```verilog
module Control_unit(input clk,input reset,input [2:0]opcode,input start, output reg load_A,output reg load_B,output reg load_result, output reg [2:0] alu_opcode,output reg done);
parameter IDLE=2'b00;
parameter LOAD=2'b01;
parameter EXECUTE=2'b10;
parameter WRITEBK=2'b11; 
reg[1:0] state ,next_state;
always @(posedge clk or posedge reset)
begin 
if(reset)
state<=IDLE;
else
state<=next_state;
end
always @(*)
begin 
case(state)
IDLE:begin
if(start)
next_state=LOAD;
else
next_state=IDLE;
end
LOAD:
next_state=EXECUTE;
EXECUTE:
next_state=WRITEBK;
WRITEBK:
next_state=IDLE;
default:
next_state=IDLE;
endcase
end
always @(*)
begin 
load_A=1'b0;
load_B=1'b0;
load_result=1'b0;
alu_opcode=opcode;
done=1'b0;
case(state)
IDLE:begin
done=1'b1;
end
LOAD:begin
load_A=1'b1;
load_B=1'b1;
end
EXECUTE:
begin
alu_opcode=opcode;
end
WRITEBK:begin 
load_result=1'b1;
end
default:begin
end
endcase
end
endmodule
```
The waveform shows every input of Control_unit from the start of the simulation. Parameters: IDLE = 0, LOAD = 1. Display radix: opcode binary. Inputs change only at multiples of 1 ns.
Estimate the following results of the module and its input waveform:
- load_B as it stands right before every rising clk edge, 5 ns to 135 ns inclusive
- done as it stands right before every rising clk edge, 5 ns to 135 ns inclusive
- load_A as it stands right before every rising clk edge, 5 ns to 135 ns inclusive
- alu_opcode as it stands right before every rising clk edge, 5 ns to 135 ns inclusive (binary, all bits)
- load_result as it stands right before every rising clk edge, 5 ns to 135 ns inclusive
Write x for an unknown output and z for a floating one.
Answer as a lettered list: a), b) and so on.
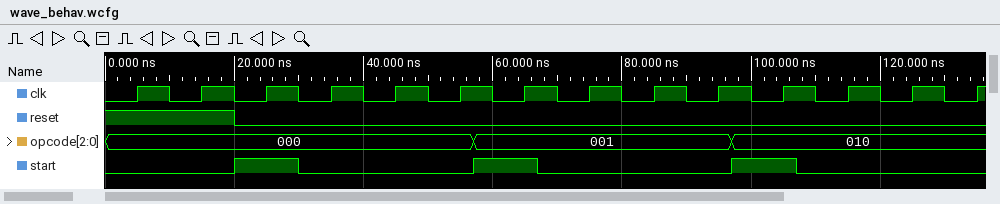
a) 0 0 0 1 0 0 0 1 0 0 0 1 0 0
b) 1 1 1 0 0 0 1 0 0 0 1 0 0 0
c) 0 0 0 1 0 0 0 1 0 0 0 1 0 0
d) 000, 000, 000, 000, 000, 000, 001, 001, 001, 001, 010, 010, 010, 010
e) 0 0 0 0 0 1 0 0 0 1 0 0 0 1
